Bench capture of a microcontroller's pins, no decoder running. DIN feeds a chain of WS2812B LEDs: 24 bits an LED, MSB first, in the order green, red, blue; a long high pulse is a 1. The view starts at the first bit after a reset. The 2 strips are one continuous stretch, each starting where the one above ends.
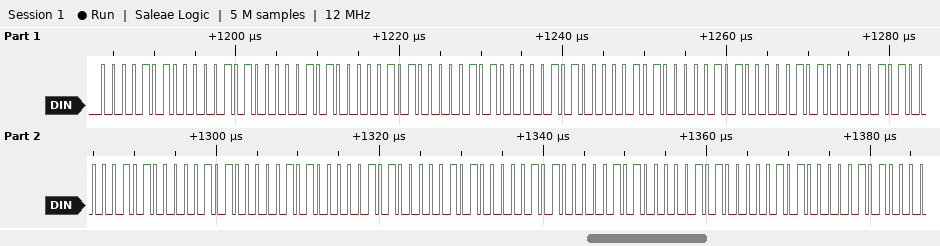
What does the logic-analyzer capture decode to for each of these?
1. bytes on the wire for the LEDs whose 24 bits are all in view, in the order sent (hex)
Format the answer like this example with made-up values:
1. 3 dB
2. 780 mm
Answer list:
1. 0A 0A 0A 0A 0A 0A 0A 0A 0A 0A 0A 0A 0A 0A 0A 0A 0A 0A
